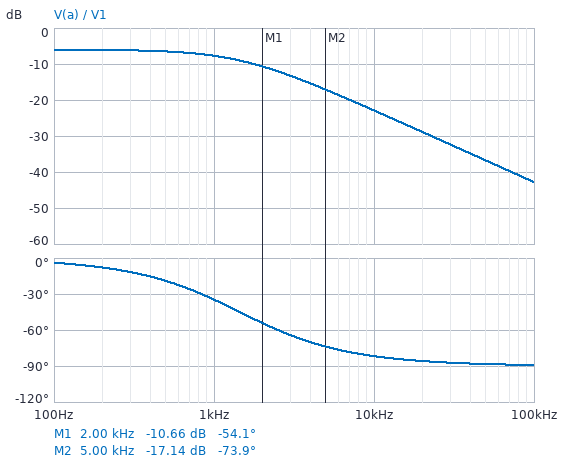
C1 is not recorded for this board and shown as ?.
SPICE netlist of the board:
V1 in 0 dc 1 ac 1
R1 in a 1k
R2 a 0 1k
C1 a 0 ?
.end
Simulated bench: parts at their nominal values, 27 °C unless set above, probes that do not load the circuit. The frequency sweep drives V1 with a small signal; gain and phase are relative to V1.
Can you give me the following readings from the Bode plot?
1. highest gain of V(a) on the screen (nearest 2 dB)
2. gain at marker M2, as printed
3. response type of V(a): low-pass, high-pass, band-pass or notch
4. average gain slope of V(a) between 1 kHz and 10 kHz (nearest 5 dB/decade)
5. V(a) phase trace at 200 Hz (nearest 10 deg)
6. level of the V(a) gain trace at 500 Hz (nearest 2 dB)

-6 dB
-17.14 dB
low-pass
-15 dB/decade
-10 deg
-6 dB
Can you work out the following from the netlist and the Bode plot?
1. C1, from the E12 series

220 nF
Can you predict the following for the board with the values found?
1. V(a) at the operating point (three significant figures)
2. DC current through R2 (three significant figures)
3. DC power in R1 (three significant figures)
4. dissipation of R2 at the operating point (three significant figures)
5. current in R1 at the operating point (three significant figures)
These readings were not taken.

500 mV
500 µA
250 µW
250 µW
500 µA
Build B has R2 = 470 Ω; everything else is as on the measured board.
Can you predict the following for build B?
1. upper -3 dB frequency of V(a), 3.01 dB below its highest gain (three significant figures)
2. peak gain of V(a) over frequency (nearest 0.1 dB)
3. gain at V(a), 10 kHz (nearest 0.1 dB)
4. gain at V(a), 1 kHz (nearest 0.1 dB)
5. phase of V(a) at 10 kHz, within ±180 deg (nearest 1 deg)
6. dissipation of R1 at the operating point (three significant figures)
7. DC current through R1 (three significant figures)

2.26 kHz
-9.9 dB
-23.0 dB
-10.7 dB
-77 deg
463 µW
680 µA
